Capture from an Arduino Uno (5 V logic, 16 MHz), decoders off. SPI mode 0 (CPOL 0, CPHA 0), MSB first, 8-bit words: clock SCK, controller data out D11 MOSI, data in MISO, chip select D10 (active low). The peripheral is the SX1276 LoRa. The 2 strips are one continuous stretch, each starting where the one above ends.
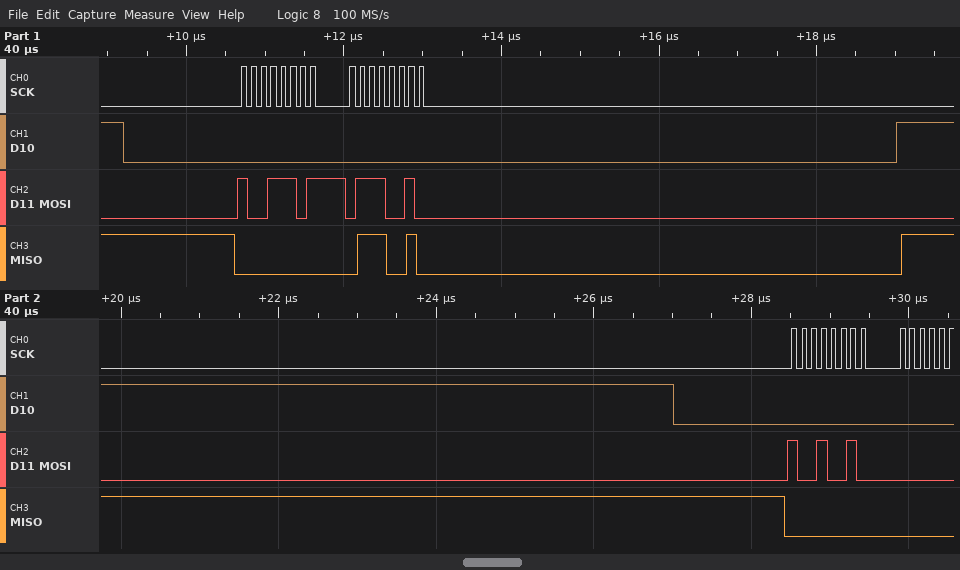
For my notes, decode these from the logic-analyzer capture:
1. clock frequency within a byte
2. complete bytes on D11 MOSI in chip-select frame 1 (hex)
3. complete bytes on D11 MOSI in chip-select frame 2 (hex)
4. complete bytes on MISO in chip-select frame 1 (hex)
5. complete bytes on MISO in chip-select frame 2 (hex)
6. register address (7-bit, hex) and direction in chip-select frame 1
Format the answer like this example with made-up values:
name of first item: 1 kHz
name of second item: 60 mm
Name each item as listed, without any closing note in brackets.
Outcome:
clock frequency within a byte: 8 MHz
complete bytes on D11 MOSI in chip-select frame 1: 0x9D 0x72
complete bytes on D11 MOSI in chip-select frame 2: 0x92
complete bytes on MISO in chip-select frame 1: 0x00 0x72
complete bytes on MISO in chip-select frame 2: 0x00
register address (7-bit, hex) and direction in chip-select frame 1: 0x1D write
